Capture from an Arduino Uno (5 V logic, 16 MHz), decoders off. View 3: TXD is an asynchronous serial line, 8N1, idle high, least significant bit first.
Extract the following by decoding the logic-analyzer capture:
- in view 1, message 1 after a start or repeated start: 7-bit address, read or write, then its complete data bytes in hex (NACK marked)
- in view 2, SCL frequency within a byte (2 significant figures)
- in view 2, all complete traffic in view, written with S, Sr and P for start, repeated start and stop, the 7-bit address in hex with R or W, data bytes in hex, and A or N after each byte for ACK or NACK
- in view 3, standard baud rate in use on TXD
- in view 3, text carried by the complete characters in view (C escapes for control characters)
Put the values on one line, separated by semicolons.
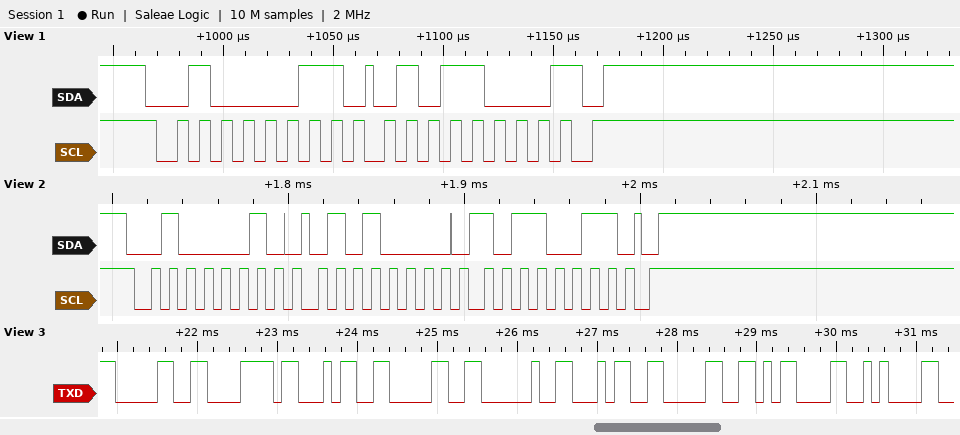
0x21 read: 58 NACK; 100 kHz; S 21W A 50 A B3 A P; 9600 baud; "0x40 40\r\n"
